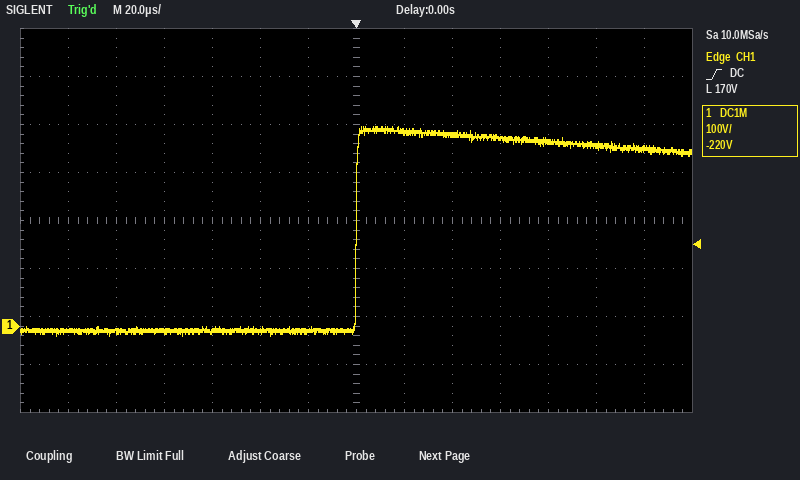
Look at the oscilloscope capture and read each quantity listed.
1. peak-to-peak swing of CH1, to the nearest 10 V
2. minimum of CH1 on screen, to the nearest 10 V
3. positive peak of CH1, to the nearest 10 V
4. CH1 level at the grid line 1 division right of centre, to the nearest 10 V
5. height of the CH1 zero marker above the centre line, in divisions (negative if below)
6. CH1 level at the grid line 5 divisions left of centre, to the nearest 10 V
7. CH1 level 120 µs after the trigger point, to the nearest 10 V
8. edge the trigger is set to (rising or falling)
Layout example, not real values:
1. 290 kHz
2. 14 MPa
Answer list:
1. 440 V
2. -20 V
3. 420 V
4. 410 V
5. -2.2 div
6. -10 V
7. 370 V
8. rising
